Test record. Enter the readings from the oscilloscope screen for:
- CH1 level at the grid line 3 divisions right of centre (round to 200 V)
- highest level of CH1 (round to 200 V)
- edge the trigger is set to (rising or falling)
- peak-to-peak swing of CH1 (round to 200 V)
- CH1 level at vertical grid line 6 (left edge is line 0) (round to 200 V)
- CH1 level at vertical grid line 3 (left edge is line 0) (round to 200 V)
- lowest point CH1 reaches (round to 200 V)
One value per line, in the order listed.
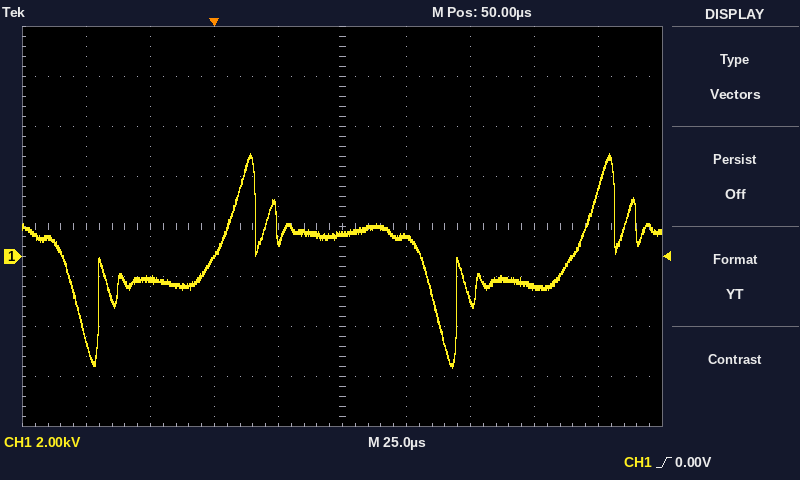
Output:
-1.2 kV
4.2 kV
rising
8.6 kV
800 V
0.0 kV
-4.4 kV
